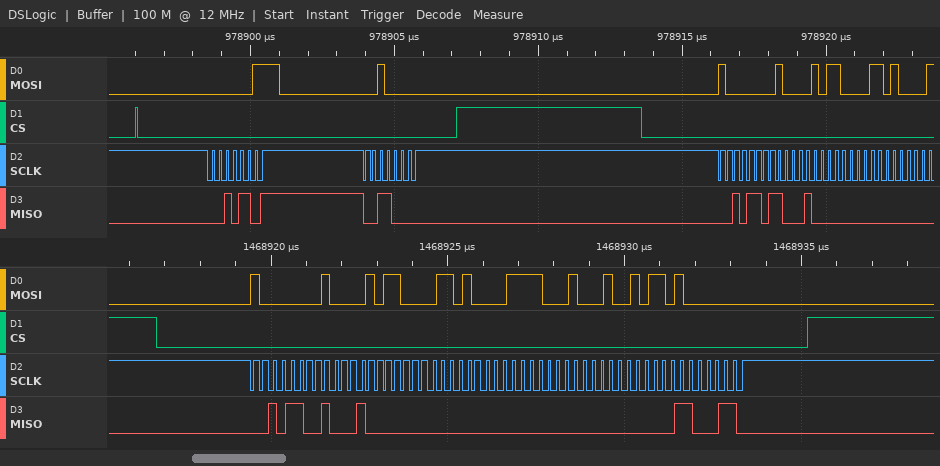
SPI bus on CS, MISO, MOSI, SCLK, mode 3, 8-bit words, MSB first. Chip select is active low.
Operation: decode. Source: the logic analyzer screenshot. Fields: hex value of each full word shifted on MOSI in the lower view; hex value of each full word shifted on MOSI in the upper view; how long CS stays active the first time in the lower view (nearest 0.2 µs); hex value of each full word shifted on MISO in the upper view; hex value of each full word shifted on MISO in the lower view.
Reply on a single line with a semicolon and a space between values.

80, 85, 86, 87, 88, 96, 80; 03, 20, 80, 85, 86; 18.4 µs; 2D, 30, 2D, 88, 00; 2C, 88, 00, 00, 00, 00, C6
